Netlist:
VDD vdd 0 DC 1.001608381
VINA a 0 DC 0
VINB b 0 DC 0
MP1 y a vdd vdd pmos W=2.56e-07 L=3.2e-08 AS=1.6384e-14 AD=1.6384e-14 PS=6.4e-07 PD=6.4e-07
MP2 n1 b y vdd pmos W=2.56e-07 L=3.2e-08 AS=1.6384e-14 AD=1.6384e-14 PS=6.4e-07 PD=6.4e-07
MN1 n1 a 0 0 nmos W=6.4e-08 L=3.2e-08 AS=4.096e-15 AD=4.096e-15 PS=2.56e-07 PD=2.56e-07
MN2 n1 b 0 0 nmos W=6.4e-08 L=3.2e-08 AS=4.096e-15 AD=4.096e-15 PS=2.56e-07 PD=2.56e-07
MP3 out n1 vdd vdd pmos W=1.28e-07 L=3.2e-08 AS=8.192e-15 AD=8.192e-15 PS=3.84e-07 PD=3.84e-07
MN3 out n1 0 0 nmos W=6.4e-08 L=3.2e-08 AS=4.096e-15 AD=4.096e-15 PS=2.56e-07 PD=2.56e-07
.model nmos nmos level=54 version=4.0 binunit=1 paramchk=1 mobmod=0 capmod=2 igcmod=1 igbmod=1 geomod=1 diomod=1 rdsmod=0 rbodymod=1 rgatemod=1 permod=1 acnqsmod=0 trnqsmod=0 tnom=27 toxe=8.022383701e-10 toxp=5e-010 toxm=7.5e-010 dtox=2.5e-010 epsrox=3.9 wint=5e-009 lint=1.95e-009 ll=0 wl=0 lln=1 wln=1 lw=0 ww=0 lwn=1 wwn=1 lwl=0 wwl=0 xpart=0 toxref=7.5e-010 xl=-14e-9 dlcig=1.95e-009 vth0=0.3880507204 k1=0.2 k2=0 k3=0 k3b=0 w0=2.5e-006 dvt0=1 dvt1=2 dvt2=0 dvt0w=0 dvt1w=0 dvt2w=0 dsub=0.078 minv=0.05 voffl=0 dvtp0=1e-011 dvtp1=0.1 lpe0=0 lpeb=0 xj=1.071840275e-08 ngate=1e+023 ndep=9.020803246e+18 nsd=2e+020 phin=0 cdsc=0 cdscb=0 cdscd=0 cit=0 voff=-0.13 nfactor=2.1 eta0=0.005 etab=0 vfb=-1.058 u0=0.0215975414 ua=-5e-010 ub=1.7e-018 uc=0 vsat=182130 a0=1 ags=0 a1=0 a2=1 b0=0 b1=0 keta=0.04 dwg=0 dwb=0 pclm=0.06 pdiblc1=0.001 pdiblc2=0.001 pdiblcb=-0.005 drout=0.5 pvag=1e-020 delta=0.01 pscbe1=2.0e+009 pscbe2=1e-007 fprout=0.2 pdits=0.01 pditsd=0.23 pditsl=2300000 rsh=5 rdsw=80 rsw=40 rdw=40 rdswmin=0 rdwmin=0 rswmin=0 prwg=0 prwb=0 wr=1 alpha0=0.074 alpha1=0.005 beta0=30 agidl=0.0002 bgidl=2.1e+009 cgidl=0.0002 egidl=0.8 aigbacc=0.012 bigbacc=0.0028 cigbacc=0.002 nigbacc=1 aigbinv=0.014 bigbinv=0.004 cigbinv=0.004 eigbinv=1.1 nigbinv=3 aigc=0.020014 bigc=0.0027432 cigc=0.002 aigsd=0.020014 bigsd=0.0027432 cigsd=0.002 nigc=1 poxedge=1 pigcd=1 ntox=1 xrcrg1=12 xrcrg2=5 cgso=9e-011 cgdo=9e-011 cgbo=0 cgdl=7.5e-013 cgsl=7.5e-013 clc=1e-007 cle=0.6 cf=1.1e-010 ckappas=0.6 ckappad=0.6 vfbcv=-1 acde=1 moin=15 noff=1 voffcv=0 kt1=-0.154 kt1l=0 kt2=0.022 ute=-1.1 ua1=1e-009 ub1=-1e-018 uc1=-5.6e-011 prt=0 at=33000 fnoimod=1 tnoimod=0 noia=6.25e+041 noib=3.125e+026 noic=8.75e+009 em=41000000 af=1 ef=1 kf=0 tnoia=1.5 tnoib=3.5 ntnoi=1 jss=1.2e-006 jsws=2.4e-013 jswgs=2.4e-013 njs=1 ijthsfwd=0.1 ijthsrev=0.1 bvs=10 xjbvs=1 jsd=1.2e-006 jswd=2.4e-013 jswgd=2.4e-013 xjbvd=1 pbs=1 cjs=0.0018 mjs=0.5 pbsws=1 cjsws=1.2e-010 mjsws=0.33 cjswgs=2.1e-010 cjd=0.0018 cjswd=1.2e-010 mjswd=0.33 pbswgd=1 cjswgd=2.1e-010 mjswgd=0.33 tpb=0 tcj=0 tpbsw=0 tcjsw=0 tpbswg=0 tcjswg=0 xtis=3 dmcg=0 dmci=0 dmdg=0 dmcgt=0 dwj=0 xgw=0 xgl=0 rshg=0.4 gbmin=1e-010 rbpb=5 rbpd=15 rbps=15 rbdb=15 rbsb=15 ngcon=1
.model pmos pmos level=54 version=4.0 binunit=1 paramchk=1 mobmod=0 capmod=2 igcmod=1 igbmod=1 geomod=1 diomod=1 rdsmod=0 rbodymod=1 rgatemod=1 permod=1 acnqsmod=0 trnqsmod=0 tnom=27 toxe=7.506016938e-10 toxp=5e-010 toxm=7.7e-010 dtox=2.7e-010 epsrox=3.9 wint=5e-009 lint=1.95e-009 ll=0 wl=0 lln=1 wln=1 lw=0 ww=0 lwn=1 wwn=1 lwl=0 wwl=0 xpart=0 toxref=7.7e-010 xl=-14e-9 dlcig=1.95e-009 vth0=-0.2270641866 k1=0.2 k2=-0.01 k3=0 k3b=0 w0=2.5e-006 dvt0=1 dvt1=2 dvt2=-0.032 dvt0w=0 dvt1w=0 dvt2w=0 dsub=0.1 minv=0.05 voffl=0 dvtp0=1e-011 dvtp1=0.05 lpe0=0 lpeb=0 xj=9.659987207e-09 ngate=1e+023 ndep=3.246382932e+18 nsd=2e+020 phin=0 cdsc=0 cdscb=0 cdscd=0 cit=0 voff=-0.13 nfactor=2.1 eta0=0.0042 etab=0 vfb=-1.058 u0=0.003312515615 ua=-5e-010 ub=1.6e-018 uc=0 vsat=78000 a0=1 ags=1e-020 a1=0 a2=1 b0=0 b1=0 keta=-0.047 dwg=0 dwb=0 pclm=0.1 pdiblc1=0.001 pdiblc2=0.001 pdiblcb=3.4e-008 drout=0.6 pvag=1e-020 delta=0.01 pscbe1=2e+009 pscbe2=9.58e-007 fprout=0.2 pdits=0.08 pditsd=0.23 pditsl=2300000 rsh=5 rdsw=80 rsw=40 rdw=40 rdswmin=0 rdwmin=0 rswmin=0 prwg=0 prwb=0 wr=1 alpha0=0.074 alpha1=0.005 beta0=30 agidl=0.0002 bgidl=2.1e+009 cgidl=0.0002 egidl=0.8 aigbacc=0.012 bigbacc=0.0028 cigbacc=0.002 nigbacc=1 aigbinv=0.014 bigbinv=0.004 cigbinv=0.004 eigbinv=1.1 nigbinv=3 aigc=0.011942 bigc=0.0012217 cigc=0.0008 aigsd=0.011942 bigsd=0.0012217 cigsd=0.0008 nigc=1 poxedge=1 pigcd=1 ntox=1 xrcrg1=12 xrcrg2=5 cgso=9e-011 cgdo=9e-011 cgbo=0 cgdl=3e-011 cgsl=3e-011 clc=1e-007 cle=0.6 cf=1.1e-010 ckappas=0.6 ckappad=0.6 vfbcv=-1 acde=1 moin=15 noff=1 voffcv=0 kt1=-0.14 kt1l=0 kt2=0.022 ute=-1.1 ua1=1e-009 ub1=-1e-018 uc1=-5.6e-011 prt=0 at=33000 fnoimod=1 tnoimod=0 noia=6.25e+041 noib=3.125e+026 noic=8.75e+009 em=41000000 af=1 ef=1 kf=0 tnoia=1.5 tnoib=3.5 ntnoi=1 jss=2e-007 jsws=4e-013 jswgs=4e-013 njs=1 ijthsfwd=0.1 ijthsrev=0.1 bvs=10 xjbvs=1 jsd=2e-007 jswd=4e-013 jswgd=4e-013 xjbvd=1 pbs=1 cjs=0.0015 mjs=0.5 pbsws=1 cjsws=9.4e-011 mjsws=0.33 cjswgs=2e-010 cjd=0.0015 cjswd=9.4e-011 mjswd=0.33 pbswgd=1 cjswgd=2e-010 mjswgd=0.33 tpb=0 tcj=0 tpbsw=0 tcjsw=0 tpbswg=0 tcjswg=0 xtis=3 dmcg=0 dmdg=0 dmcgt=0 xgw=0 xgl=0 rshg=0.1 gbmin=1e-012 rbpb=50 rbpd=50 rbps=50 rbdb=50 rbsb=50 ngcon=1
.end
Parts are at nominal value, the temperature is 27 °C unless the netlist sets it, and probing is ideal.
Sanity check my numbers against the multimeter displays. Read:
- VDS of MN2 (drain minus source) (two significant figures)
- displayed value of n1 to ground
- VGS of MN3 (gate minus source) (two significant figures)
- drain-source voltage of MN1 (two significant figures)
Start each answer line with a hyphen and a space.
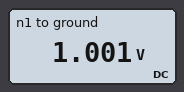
- 1.0 V
- 1.001 V
- 1.0 V
- 1.0 V
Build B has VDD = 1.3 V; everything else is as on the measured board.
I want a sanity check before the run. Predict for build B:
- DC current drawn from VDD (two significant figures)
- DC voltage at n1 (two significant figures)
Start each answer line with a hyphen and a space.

- 3.2 µA
- 1.3 V
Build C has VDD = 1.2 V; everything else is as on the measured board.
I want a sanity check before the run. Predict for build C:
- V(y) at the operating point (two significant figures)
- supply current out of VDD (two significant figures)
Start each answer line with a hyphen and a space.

- 1.2 V
- 1.5 µA
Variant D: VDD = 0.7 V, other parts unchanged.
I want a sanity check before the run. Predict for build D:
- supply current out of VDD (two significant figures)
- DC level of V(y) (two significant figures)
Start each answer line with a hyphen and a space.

- 170 nA
- 700 mV
